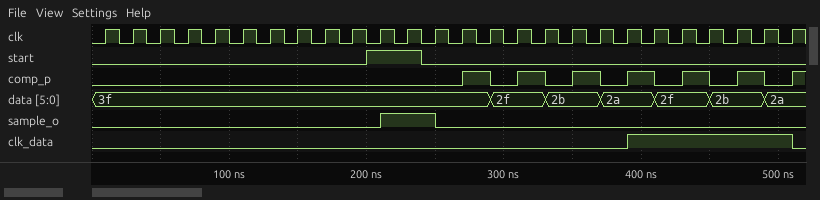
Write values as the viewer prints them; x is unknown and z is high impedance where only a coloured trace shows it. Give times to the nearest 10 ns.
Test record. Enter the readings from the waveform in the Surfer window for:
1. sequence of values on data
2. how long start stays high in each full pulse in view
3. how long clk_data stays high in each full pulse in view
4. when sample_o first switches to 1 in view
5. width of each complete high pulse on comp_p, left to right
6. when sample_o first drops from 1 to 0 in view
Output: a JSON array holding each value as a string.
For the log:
["3f, 2f, 2b, 2a, 2f, 2b, 2a", "40 ns", "120 ns", "210 ns", "20 ns, 20 ns, 20 ns, 20 ns, 20 ns, 20 ns", "250 ns"]
